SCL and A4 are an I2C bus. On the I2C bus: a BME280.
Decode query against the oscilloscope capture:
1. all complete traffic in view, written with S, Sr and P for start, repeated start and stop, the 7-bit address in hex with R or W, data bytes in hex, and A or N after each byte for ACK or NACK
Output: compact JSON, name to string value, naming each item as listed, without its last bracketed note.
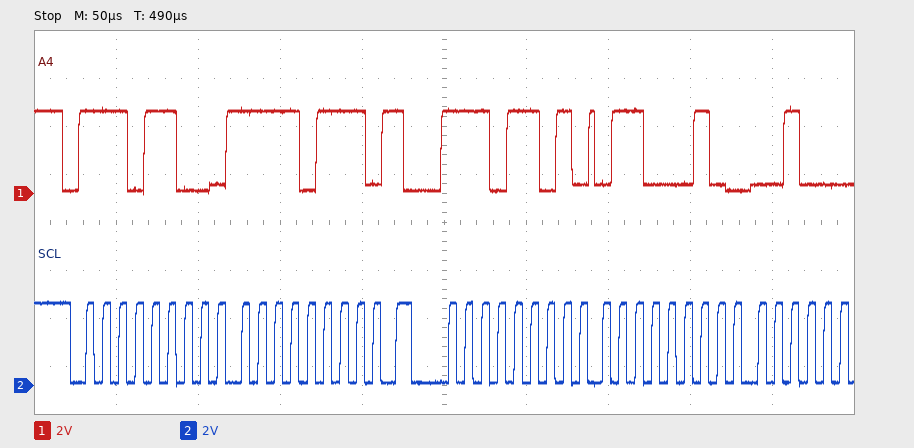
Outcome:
{"all complete traffic in view, written with S, Sr and P for start, repeated start and stop, the 7-bit address in hex with R or W, data bytes in hex, and A or N after each byte for ACK or NACK": "S 76W A F7 A Sr 76R A 62 A"}
